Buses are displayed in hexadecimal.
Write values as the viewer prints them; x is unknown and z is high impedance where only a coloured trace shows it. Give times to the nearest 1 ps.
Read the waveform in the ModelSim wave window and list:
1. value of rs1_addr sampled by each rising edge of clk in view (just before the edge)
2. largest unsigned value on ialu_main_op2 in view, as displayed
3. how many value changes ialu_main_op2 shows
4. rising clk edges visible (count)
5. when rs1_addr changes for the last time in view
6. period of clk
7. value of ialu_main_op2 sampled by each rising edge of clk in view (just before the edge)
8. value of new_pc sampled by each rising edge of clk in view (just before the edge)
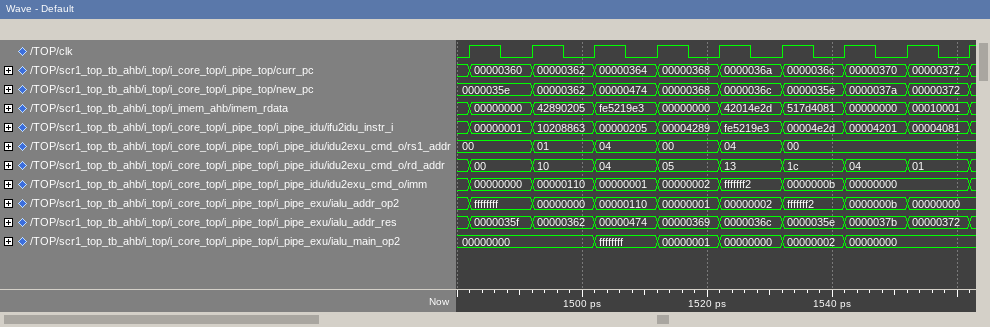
00, 00, 01, 04, 00, 04, 00, 00, 00
ffffffff
5
9
1532 ps
10 ps
00000000, 00000000, 00000000, ffffffff, 00000001, 00000000, 00000002, 00000000, 00000000
0000035e, 0000035e, 00000362, 00000474, 00000368, 0000036c, 0000035e, 0000037a, 00000372
